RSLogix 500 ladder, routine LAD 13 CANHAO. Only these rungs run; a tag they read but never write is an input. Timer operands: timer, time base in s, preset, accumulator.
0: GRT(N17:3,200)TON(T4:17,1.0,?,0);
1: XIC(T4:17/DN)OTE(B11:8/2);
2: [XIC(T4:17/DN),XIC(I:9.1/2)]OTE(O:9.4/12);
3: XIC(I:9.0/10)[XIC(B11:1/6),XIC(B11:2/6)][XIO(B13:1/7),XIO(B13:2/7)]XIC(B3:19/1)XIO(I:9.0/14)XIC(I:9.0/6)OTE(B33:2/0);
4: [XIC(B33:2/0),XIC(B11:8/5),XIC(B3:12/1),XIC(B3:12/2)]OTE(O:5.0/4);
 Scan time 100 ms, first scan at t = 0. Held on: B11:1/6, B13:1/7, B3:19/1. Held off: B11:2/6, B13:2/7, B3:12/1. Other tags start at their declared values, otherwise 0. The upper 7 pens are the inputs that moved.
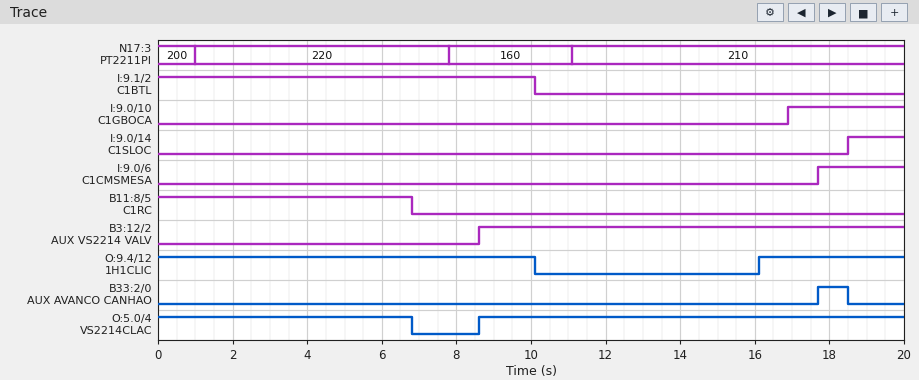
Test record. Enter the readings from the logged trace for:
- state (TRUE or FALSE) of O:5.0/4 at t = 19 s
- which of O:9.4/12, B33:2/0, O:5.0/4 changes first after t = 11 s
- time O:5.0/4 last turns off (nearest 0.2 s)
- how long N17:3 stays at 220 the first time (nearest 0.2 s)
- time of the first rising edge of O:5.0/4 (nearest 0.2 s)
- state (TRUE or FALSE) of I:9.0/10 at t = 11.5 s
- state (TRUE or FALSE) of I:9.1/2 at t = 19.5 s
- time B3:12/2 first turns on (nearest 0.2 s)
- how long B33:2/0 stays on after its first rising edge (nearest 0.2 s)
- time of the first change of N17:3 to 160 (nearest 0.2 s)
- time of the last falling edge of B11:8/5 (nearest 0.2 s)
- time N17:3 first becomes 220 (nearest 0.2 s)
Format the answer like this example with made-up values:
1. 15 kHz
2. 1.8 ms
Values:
1. TRUE
2. O:9.4/12
3. 6.8 s
4. 6.8 s
5. 8.6 s
6. FALSE
7. FALSE
8. 8.6 s
9. 0.8 s
10. 7.8 s
11. 6.8 s
12. 1.0 s
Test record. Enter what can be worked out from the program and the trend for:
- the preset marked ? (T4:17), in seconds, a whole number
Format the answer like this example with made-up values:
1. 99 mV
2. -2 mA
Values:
1. 5 s
